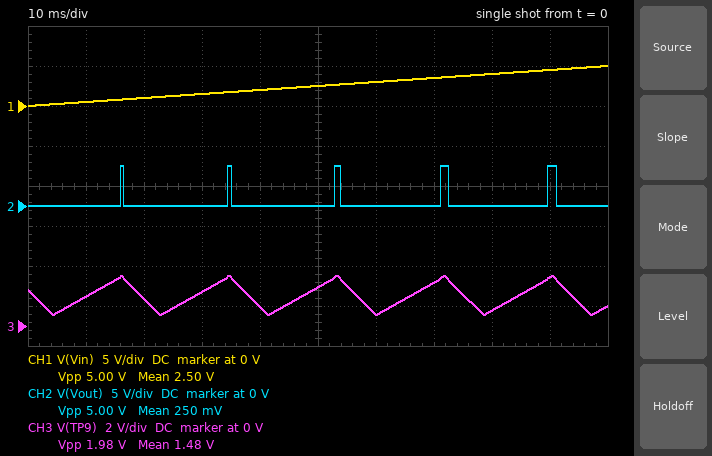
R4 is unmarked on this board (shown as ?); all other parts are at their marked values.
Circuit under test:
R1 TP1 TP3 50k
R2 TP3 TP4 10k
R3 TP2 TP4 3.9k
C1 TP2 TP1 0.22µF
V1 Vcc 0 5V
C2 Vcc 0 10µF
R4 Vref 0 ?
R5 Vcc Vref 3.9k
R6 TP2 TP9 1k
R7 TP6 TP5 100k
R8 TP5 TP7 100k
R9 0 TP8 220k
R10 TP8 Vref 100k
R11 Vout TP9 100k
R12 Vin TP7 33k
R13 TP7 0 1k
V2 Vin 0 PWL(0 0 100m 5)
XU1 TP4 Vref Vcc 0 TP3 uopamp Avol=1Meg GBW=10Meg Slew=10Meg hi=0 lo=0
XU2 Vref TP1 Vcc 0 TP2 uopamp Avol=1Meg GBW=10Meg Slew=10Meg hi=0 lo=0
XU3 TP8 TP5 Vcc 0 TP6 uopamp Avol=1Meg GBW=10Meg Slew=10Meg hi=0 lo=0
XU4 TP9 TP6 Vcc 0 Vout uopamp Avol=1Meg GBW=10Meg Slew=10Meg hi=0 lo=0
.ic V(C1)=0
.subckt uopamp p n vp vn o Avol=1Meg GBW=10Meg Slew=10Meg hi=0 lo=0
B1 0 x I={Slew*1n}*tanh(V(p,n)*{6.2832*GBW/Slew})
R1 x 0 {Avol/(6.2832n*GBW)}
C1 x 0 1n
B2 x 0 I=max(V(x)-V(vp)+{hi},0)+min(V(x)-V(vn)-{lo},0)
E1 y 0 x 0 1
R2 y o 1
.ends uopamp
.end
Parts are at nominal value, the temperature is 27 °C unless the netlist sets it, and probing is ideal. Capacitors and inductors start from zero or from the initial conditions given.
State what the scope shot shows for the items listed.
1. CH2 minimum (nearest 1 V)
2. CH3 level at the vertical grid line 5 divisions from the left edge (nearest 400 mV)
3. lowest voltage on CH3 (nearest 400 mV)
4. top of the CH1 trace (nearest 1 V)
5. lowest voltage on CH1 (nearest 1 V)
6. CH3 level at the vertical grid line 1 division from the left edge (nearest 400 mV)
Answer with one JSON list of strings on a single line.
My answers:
["0 V", "2.0 V", "400 mV", "5 V", "0 V", "1.6 V"]
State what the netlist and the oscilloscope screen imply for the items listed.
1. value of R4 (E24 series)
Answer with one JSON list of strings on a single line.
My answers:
["2.2 kΩ"]
